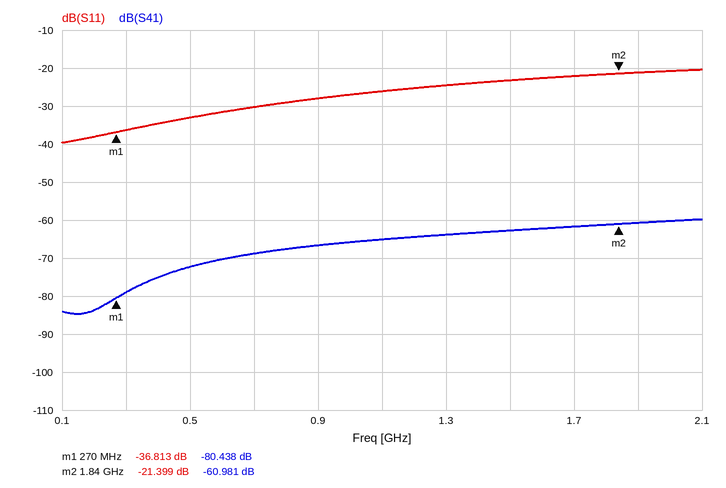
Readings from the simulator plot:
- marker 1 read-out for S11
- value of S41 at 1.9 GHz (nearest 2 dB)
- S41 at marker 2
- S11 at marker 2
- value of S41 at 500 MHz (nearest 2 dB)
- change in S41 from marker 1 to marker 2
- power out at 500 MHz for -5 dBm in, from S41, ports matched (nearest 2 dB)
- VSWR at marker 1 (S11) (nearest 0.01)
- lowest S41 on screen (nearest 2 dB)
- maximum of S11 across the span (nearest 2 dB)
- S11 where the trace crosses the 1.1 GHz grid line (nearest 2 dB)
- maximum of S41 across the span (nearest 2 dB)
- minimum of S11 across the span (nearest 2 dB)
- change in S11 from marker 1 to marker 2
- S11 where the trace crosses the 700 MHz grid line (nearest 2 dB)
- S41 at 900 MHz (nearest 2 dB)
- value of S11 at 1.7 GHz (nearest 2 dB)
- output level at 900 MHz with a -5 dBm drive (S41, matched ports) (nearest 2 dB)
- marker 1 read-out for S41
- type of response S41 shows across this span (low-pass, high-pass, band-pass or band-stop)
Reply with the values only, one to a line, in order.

-36.813 dB
-60 dB
-60.981 dB
-21.399 dB
-72 dB
19.457 dB
-78 dBm
1.03
-84 dB
-20 dB
-26 dB
-60 dB
-40 dB
15.414 dB
-30 dB
-66 dB
-22 dB
-72 dBm
-80.438 dB
high-pass
